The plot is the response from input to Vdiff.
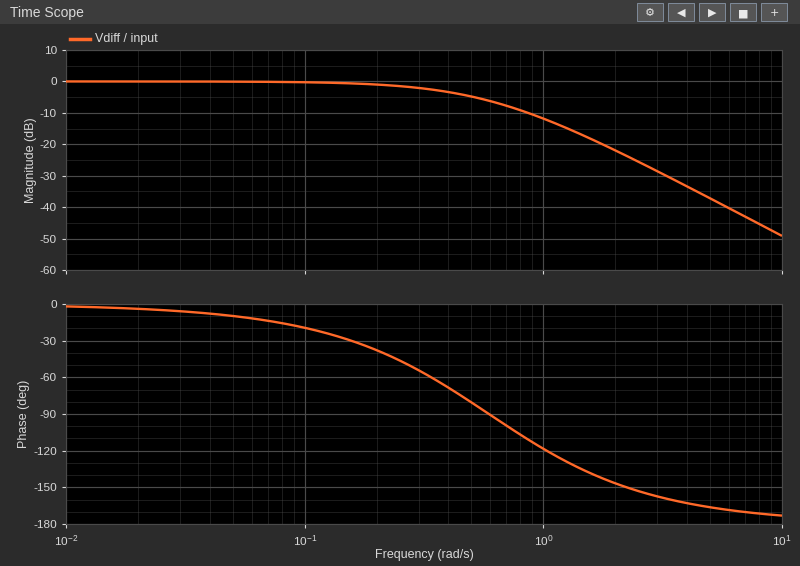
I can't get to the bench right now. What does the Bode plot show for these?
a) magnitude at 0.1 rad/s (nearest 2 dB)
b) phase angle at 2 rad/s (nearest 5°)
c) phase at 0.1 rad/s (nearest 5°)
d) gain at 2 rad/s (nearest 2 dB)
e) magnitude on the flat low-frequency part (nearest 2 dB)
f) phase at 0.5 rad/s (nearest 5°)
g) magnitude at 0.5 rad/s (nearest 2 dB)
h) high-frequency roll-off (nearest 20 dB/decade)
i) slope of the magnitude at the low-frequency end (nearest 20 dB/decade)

0 dB
-145°
-20°
-22 dB
0 dB
-80°
-4 dB
-40 dB/decade
0 dB/decade
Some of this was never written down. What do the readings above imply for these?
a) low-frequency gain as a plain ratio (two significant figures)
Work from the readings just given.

1.0
